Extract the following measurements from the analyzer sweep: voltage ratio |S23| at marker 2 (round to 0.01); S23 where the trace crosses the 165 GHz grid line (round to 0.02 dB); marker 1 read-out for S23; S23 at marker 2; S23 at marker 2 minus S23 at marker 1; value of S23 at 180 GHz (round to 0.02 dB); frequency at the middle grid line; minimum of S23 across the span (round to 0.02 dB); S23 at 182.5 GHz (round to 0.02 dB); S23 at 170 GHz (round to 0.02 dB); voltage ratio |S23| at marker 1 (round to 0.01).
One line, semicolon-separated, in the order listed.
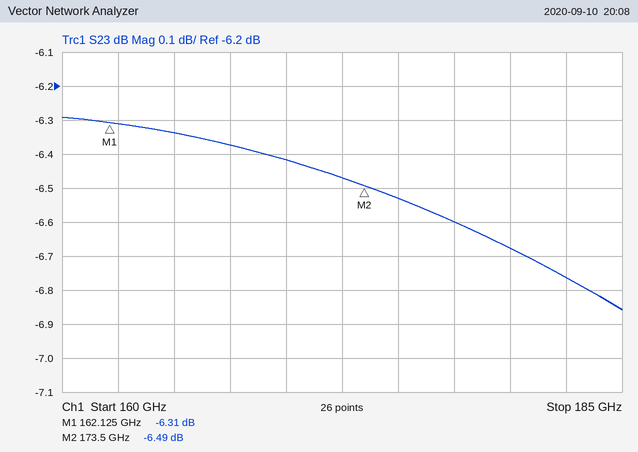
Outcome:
0.47; -6.34 dB; -6.31 dB; -6.49 dB; -0.18 dB; -6.68 dB; 172.5 GHz; -6.86 dB; -6.76 dB; -6.42 dB; 0.48
